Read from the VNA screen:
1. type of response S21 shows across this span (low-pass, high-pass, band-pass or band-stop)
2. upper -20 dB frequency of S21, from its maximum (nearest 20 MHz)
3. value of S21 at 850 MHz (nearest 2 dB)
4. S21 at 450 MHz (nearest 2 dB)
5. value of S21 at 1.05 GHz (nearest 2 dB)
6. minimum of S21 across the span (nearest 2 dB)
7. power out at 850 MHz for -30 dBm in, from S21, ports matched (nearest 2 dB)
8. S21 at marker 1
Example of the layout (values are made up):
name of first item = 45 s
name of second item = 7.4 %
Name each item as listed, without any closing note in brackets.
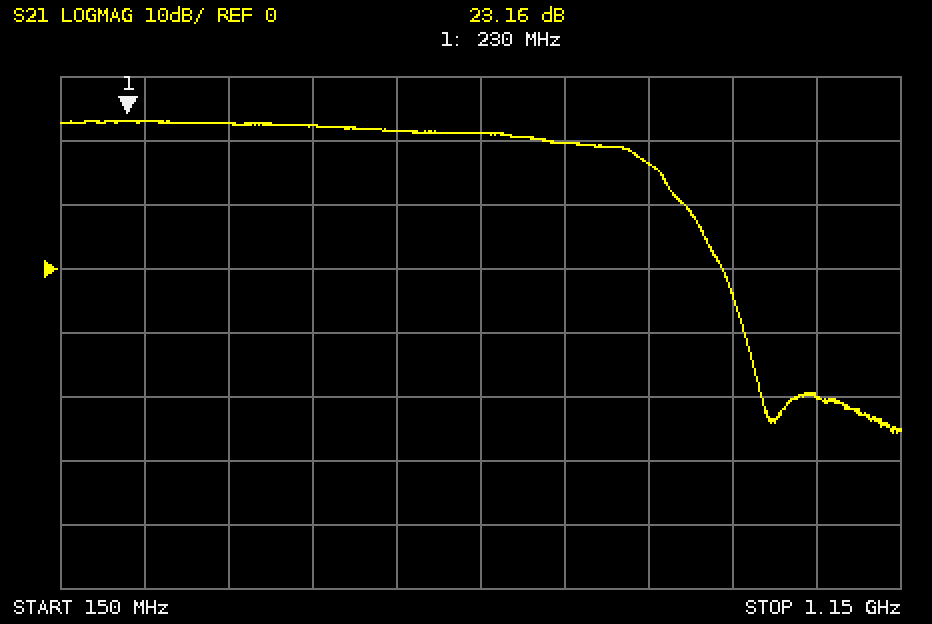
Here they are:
type of response S21 shows across this span = low-pass
upper -20 dB frequency of S21, from its maximum = 920 MHz
value of S21 at 850 MHz = 16 dB
S21 at 450 MHz = 22 dB
value of S21 at 1.05 GHz = -20 dB
minimum of S21 across the span = -26 dB
power out at 850 MHz for -30 dBm in, from S21, ports matched = -14 dBm
S21 at marker 1 = 23.16 dB
